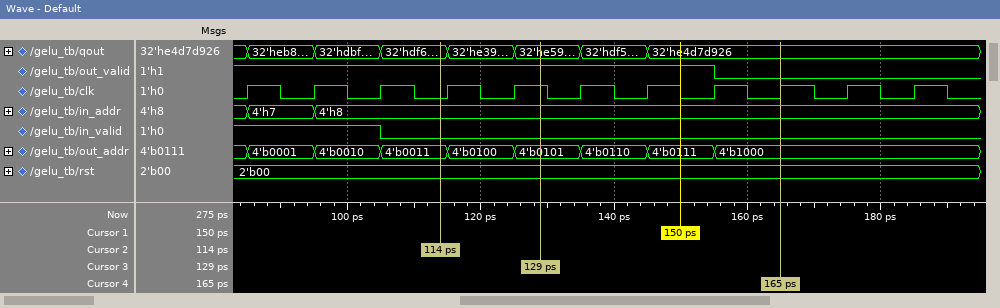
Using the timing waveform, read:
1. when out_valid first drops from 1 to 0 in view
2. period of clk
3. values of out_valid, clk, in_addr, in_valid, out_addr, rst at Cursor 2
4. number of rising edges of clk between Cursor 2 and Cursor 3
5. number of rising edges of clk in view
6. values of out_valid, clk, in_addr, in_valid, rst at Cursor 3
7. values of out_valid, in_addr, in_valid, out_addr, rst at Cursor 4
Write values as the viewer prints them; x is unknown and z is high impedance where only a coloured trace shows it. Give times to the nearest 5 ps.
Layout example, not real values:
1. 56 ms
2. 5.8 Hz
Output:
1. 155 ps
2. 10 ps
3. out_valid=1, clk=0, in_addr=4'h8, in_valid=0, out_addr=4'b0011, rst=2'b00
4. 2
5. 11
6. out_valid=1, clk=1, in_addr=4'h8, in_valid=0, rst=2'b00
7. out_valid=0, in_addr=4'h8, in_valid=0, out_addr=4'b1000, rst=2'b00
